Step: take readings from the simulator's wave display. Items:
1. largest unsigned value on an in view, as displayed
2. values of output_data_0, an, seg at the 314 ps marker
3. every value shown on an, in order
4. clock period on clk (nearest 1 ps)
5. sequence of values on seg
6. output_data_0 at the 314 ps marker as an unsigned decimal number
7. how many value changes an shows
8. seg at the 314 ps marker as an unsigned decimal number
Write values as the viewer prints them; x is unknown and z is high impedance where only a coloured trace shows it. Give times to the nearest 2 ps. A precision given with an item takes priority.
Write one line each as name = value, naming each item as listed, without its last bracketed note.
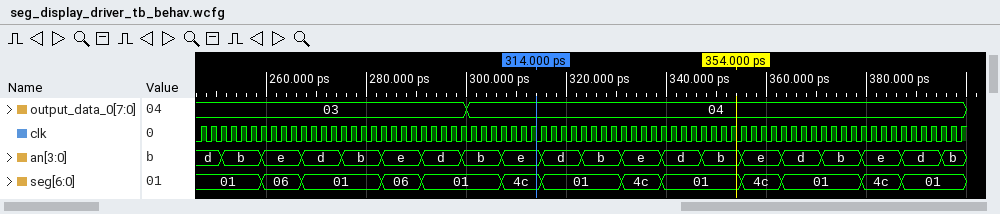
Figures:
largest unsigned value on an in view, as displayed = e
values of output_data_0, an, seg at the 314 ps marker = output_data_0=04, an=e, seg=4c
every value shown on an, in order = d, b, e, d, b, e, d, b, e, d, b, e, d, b, e, d, b, e, d, b
clock period on clk = 2 ps
sequence of values on seg = 01, 06, 01, 06, 01, 4c, 01, 4c, 01, 4c, 01, 4c, 01
output_data_0 at the 314 ps marker as an unsigned decimal number = 4
how many value changes an shows = 19
seg at the 314 ps marker as an unsigned decimal number = 76
